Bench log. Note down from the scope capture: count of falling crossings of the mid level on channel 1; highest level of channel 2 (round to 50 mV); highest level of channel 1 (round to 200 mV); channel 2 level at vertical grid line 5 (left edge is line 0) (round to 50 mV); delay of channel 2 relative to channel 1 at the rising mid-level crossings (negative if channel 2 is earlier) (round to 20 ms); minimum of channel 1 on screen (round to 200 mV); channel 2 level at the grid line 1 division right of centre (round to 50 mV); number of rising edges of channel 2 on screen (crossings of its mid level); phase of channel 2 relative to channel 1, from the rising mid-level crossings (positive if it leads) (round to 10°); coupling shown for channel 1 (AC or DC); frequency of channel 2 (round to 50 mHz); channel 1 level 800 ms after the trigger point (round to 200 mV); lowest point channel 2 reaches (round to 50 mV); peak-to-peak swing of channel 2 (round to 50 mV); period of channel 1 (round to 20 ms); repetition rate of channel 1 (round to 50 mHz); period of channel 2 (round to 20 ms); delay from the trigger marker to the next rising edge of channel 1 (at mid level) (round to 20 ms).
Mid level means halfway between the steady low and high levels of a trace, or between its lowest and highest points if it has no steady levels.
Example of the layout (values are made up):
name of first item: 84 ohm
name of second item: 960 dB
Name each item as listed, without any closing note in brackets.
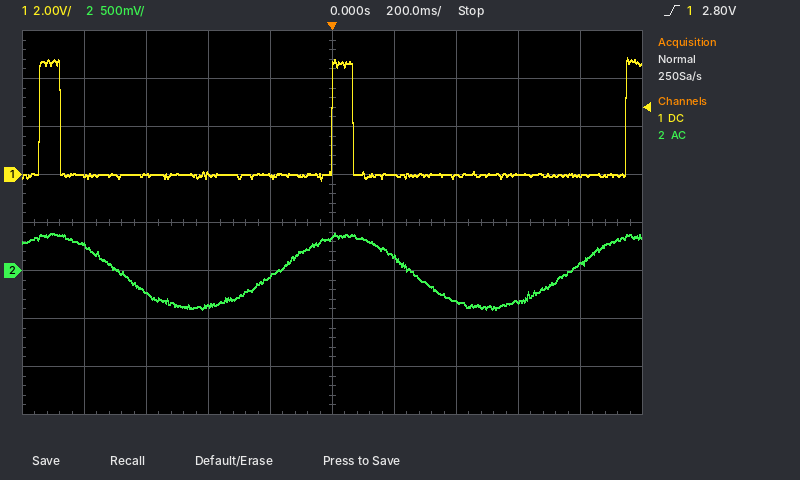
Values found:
count of falling crossings of the mid level on channel 1: 2
highest level of channel 2: 400 mV
highest level of channel 1: 4.8 V
channel 2 level at vertical grid line 5 (left edge is line 0): 350 mV
delay of channel 2 relative to channel 1 at the rising mid-level crossings (negative if channel 2 is earlier): -180 ms
minimum of channel 1 on screen: -200 mV
channel 2 level at the grid line 1 division right of centre: 150 mV
number of rising edges of channel 2 on screen: 2
phase of channel 2 relative to channel 1, from the rising mid-level crossings (positive if it leads): +70°
coupling shown for channel 1: DC
frequency of channel 2: 1.05 Hz
channel 1 level 800 ms after the trigger point: 0.0 V
lowest point channel 2 reaches: -400 mV
peak-to-peak swing of channel 2: 800 mV
period of channel 1: 940 ms
repetition rate of channel 1: 1.05 Hz
period of channel 2: 940 ms
delay from the trigger marker to the next rising edge of channel 1 (at mid level): 940 ms
